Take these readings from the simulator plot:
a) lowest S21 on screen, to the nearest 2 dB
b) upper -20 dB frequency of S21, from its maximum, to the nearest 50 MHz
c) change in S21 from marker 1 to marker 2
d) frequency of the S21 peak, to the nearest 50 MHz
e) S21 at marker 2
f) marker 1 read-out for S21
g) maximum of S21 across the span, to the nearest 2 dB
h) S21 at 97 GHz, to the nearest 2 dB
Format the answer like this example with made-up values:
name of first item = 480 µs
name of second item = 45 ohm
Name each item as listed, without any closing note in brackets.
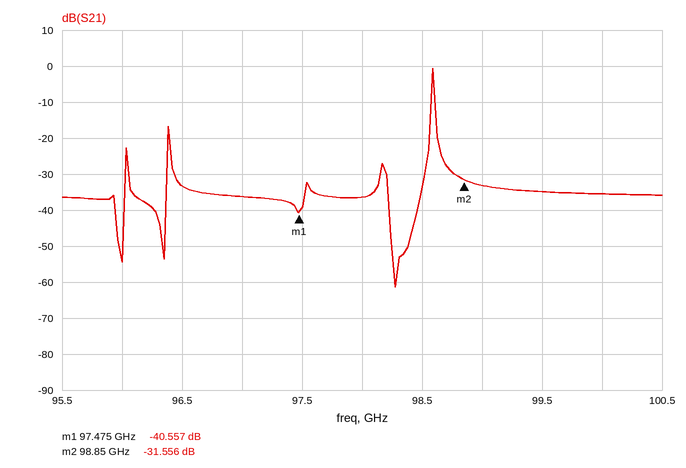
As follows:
lowest S21 on screen, to the nearest 2 dB = -62 dB
upper -20 dB frequency of S21, from its maximum, to the nearest 50 MHz = 98.65 GHz
change in S21 from marker 1 to marker 2 = 9.001 dB
frequency of the S21 peak, to the nearest 50 MHz = 98.60 GHz
S21 at marker 2 = -31.556 dB
marker 1 read-out for S21 = -40.557 dB
maximum of S21 across the span, to the nearest 2 dB = 0 dB
S21 at 97 GHz, to the nearest 2 dB = -36 dB
